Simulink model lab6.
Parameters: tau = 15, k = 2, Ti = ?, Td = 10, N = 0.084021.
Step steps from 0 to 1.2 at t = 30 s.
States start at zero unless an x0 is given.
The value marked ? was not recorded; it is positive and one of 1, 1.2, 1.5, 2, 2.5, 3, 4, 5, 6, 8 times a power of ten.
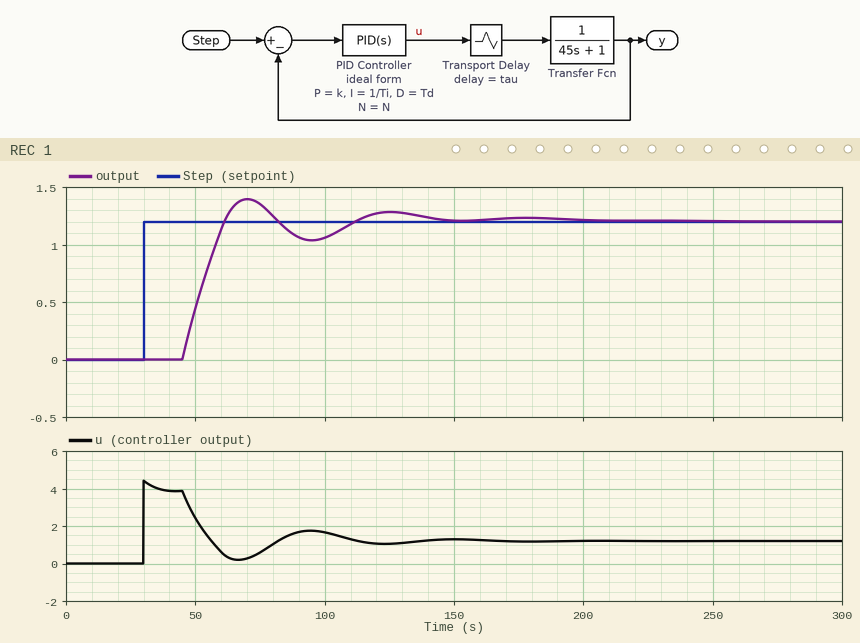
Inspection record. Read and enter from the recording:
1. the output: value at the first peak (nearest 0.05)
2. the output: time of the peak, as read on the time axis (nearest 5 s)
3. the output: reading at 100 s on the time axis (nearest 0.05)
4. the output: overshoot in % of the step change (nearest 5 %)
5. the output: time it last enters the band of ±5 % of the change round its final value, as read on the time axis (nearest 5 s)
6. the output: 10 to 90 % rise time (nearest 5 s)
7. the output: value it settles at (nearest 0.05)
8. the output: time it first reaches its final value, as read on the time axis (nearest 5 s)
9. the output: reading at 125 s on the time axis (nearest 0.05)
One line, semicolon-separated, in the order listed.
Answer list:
1.40; 70 s; 1.05; 15 %; 135 s; 15 s; 1.20; 60 s; 1.30
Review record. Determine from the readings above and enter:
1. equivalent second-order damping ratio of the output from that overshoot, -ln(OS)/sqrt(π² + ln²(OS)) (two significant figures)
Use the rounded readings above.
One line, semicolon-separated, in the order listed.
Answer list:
0.52
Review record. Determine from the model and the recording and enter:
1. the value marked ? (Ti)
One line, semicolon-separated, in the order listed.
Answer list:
40
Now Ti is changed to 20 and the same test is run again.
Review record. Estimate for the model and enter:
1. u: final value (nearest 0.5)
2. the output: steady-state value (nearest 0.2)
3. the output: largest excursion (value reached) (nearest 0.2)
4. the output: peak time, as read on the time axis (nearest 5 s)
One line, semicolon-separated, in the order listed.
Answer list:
1.0; 1.2; 1.8; 75 s
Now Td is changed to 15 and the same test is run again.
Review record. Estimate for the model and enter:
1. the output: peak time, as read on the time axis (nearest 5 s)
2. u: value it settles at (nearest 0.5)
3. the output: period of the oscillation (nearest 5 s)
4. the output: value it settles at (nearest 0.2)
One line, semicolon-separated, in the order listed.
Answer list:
65 s; 1.0; 50 s; 1.2
